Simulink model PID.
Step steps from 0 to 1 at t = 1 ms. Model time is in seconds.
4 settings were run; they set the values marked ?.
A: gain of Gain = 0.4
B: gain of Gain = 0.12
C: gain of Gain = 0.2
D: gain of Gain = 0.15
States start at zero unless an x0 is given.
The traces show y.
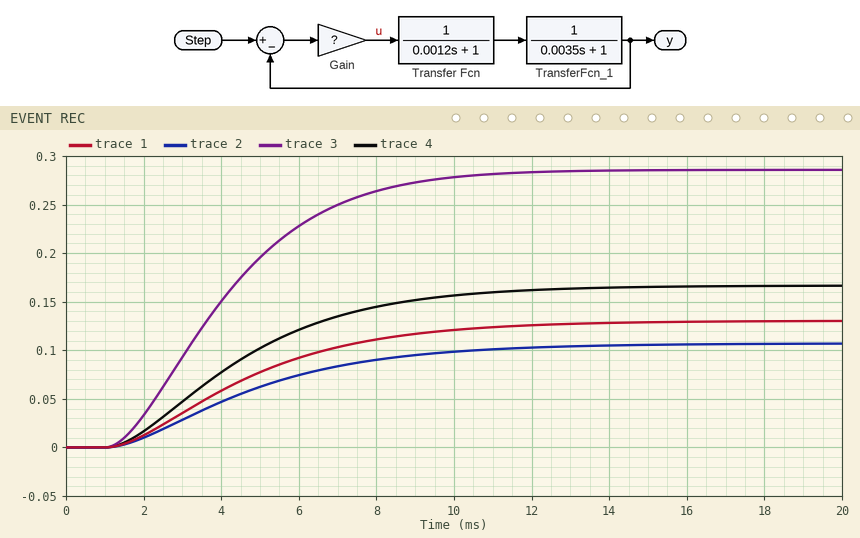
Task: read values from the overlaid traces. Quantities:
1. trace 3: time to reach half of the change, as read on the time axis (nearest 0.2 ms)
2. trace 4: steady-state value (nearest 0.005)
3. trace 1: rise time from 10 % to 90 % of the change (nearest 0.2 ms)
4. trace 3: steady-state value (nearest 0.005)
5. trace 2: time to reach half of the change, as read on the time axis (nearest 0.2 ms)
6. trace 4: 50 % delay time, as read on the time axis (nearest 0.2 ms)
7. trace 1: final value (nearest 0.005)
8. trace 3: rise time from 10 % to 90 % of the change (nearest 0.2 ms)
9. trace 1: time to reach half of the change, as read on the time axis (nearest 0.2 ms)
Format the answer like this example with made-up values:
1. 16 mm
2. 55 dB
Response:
1. 3.8 ms
2. 0.165
3. 7.0 ms
4. 0.285
5. 4.4 ms
6. 4.2 ms
7. 0.130
8. 5.6 ms
9. 4.4 ms
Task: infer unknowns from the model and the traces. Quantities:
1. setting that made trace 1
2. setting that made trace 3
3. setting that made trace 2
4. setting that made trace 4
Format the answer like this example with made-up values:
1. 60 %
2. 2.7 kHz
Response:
1. D
2. A
3. B
4. C
